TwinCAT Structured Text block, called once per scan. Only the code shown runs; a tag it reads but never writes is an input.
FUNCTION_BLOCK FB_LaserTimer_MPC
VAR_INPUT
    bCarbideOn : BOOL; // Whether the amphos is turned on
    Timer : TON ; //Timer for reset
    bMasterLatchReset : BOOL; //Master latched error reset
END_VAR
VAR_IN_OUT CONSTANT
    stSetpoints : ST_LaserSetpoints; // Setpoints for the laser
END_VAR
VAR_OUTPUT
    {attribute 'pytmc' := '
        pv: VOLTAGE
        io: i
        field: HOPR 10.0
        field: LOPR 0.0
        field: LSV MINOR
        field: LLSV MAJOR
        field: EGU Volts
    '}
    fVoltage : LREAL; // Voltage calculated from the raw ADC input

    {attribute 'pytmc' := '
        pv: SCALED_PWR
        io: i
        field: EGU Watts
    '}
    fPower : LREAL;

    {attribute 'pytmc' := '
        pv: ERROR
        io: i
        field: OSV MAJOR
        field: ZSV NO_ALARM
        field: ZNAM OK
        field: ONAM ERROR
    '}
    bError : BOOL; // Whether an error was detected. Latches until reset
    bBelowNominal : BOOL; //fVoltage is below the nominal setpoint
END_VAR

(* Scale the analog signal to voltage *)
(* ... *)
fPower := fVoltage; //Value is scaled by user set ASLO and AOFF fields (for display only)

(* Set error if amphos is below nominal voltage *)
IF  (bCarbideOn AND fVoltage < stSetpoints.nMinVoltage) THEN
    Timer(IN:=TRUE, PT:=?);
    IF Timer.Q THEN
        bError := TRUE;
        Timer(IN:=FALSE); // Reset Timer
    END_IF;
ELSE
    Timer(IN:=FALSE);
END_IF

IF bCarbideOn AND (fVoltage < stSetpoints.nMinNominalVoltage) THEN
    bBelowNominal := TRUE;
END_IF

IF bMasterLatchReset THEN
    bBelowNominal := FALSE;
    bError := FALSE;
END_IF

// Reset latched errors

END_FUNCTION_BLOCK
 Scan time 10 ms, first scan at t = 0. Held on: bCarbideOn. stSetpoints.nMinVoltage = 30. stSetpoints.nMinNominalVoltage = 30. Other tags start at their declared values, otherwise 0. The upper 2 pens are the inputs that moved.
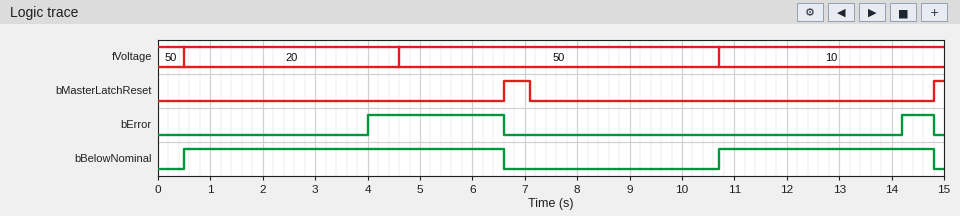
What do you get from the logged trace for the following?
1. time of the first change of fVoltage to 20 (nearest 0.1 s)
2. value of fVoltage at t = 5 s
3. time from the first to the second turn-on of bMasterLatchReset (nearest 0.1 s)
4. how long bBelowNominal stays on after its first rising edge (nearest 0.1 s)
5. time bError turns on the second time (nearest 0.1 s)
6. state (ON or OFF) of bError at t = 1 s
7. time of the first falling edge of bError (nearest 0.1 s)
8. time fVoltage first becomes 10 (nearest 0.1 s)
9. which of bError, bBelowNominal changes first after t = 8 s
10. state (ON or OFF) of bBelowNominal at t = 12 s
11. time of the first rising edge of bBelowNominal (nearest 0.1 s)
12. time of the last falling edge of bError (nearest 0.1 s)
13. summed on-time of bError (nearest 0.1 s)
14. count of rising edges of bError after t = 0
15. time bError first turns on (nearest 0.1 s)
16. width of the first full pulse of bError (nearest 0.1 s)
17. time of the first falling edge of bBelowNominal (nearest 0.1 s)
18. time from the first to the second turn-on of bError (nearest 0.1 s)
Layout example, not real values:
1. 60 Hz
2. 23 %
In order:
1. 0.5 s
2. 50
3. 8.2 s
4. 6.1 s
5. 14.2 s
6. OFF
7. 6.6 s
8. 10.7 s
9. bBelowNominal
10. ON
11. 0.5 s
12. 14.8 s
13. 3.2 s
14. 2
15. 4.0 s
16. 2.6 s
17. 6.6 s
18. 10.2 s
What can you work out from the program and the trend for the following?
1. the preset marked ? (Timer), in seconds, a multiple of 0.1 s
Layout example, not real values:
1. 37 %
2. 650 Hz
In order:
1. 3.5 s
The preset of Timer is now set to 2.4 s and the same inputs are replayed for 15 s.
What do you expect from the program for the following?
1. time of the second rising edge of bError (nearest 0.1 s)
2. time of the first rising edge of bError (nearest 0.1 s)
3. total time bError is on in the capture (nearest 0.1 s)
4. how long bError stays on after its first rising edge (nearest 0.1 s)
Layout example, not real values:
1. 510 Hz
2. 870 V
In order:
1. 13.1 s
2. 2.9 s
3. 5.4 s
4. 3.7 s
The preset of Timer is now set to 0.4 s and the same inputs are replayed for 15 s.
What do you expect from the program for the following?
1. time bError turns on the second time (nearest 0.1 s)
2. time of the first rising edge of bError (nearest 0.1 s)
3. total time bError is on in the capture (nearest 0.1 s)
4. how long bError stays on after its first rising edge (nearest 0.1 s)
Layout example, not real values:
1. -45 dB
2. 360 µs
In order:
1. 11.1 s
2. 0.9 s
3. 9.4 s
4. 5.7 s
